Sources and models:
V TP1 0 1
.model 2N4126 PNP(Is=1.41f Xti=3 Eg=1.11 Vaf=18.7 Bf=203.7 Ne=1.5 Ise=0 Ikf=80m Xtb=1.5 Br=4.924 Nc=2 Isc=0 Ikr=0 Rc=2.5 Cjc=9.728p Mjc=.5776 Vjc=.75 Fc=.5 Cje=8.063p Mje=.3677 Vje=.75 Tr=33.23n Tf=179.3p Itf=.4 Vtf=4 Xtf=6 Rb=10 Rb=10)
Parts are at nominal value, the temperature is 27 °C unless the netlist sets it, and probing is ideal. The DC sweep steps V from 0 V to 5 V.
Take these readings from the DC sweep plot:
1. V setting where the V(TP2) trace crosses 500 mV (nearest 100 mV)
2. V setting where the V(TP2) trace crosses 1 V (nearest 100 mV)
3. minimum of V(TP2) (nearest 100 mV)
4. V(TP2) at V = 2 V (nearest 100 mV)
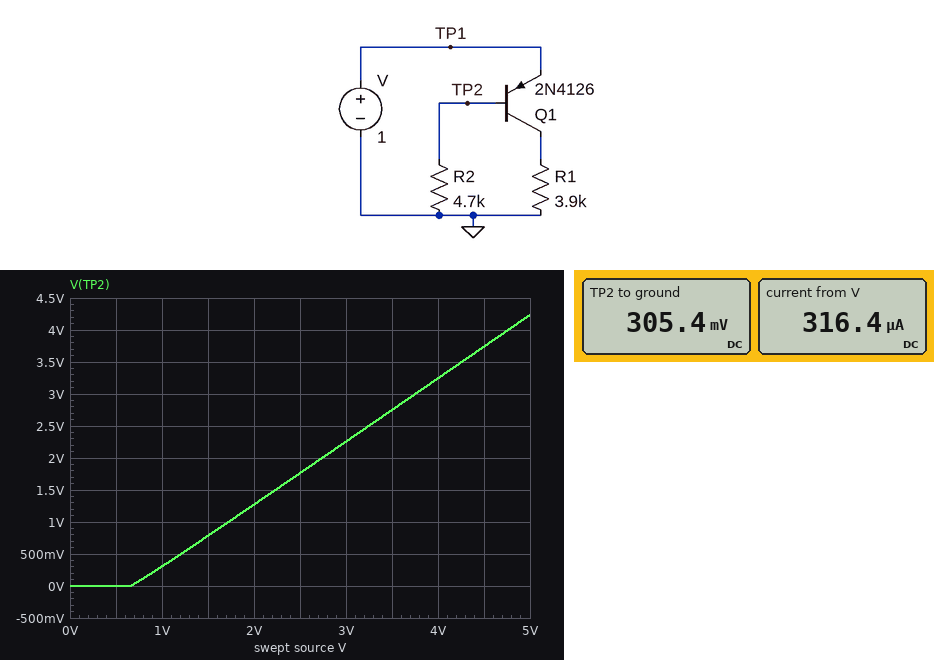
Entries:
1.2 V
1.7 V
0 V
1.3 V
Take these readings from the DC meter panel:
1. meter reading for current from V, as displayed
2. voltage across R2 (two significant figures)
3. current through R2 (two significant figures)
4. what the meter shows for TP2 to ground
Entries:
316.4 µA
310 mV
65 µA
305.4 mV
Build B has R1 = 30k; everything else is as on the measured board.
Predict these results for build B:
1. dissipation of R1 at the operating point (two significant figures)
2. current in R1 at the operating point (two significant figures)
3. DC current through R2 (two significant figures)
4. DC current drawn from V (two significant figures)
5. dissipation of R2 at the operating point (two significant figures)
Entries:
33 µW
33 µA
67 µA
100 µA
21 µW
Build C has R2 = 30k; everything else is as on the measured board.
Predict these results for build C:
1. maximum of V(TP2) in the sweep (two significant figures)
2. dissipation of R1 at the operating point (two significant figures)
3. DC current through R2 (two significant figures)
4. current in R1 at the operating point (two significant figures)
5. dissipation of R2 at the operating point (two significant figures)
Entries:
4.3 V
230 µW
11 µA
240 µA
3.5 µW
